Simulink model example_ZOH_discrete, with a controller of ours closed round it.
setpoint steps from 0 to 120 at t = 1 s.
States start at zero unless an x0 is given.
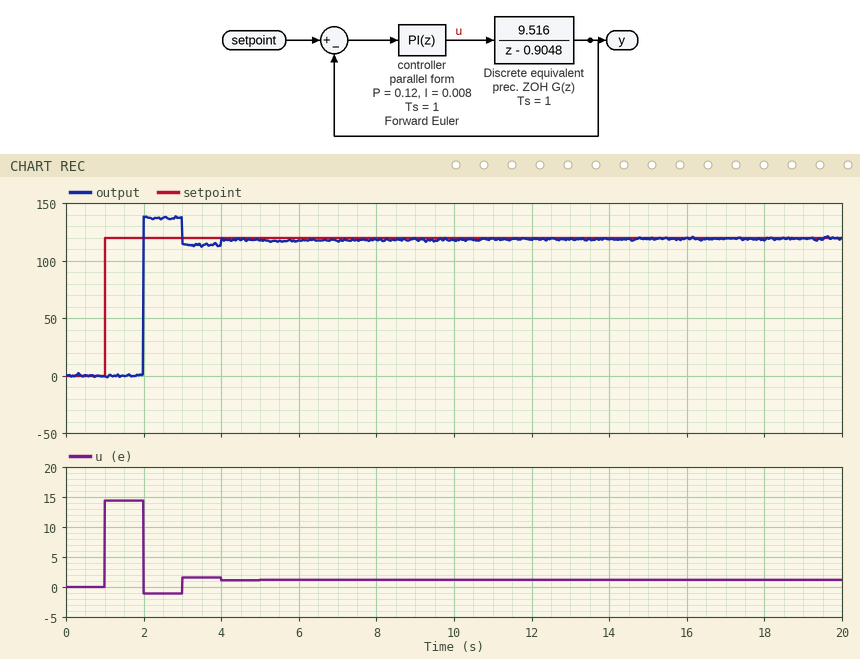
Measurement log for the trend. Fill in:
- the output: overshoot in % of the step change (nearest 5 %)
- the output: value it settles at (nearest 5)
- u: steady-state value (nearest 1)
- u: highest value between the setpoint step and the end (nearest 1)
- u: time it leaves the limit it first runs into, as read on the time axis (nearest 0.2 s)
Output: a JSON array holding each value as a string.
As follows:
["15 %", "120", "1", "14", "2.0 s"]
